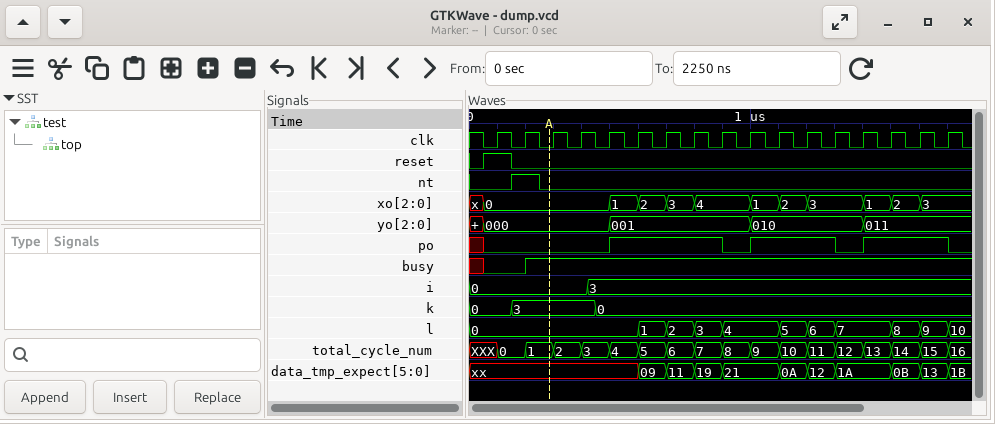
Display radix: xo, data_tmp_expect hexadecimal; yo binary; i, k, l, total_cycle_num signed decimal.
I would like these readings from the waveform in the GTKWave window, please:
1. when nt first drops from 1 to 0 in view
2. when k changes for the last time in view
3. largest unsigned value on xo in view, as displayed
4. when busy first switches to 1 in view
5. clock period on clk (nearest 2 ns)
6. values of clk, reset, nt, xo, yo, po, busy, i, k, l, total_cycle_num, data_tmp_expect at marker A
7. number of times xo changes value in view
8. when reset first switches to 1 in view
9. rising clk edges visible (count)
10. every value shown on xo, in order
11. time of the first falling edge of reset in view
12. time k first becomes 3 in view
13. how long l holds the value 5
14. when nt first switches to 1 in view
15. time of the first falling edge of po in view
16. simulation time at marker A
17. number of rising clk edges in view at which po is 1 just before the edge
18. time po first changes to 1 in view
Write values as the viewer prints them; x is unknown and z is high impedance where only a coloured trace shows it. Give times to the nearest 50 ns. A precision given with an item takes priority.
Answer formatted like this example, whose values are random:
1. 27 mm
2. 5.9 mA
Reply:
1. 250 ns
2. 450 ns
3. 4
4. 200 ns
5. 100 ns
6. clk=0, reset=0, nt=0, xo=0, yo=000, po=0, busy=1, i=0, k=3, l=0, total_cycle_num=1, data_tmp_expect=xx
7. 11
8. 50 ns
9. 17
10. x, 0, 1, 2, 3, 4, 1, 2, 3, 1, 2, 3
11. 150 ns
12. 150 ns
13. 100 ns
14. 150 ns
15. 900 ns
16. 300 ns
17. 10
18. 500 ns
